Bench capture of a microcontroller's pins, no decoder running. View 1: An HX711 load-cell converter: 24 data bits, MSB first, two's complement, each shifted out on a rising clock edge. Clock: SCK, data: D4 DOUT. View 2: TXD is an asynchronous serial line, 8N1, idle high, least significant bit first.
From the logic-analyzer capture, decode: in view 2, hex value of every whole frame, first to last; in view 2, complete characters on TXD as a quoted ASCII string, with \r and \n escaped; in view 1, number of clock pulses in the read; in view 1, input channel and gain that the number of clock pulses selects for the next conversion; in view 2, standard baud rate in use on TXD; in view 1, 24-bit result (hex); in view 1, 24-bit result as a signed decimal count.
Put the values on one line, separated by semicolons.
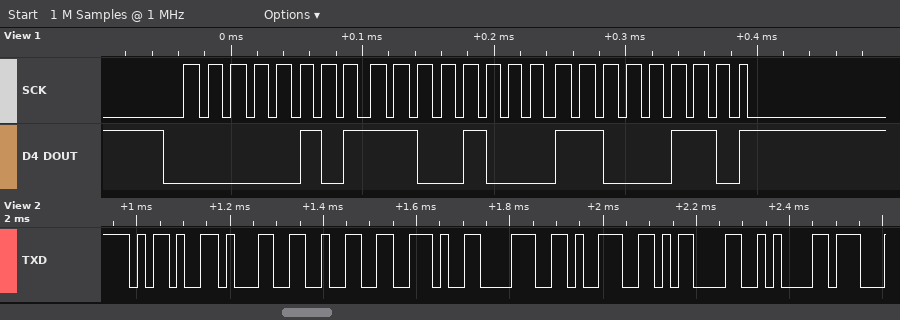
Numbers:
2D 31 32 2E 38 39 0D 0A; "-12.89\r\n"; 25; channel A, gain 128; 57600 baud; 0x05C8C6; 379078
